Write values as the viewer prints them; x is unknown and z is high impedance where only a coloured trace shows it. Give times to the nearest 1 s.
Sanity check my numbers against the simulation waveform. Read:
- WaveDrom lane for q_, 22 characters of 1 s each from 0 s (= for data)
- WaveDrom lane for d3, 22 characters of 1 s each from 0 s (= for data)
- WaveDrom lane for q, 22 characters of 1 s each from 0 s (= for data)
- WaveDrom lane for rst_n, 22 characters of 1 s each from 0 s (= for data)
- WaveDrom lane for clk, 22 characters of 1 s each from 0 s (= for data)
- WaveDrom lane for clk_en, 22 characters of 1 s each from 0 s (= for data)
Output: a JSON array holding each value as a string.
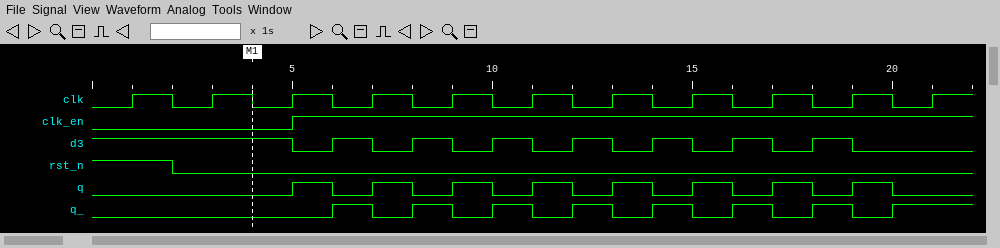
["{name: 'q_', wave: '0.....101010101010101.'}", "{name: 'd3', wave: '1....010101010101010..'}", "{name: 'q', wave: '0....1010101010101010.'}", "{name: 'rst_n', wave: '1.0...................'}", "{name: 'clk', wave: '0101010101010101010101'}", "{name: 'clk_en', wave: '0....1................'}"]
